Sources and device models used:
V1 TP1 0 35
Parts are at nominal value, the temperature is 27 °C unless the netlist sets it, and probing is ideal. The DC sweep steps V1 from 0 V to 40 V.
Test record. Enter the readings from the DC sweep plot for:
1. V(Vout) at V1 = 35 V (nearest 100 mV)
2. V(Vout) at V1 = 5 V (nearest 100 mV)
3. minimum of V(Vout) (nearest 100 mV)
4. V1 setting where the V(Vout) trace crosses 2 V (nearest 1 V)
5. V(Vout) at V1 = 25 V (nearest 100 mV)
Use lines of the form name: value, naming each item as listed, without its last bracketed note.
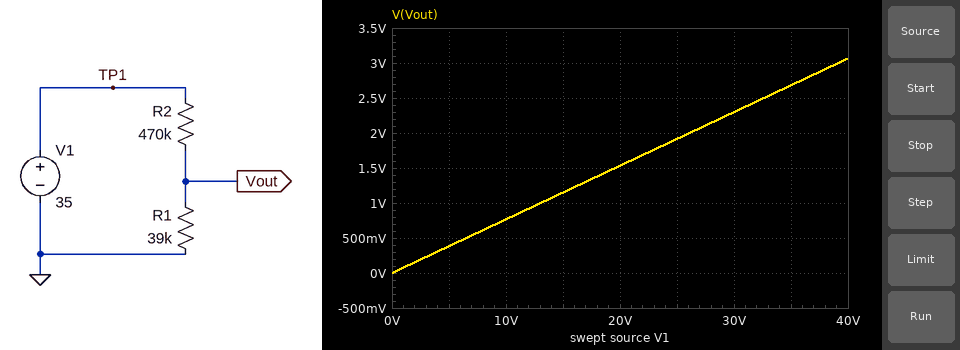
V(Vout) at V1 = 35 V: 2.7 V
V(Vout) at V1 = 5 V: 400 mV
minimum of V(Vout): 0 V
V1 setting where the V(Vout) trace crosses 2 V: 26 V
V(Vout) at V1 = 25 V: 1.9 V
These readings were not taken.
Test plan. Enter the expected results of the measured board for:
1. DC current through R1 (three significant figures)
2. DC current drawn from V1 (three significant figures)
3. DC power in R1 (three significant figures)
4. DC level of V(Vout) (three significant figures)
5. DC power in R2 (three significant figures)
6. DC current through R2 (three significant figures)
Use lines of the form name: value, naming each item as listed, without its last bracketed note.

DC current through R1: 68.8 µA
DC current drawn from V1: 68.8 µA
DC power in R1: 184 µW
DC level of V(Vout): 2.68 V
DC power in R2: 2.22 mW
DC current through R2: 68.8 µA
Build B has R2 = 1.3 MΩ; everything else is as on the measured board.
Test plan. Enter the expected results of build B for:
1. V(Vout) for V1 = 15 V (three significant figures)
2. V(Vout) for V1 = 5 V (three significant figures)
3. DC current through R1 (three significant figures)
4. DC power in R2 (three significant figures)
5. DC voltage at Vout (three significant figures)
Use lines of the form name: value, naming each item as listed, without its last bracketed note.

V(Vout) for V1 = 15 V: 437 mV
V(Vout) for V1 = 5 V: 146 mV
DC current through R1: 26.1 µA
DC power in R2: 888 µW
DC voltage at Vout: 1.02 V
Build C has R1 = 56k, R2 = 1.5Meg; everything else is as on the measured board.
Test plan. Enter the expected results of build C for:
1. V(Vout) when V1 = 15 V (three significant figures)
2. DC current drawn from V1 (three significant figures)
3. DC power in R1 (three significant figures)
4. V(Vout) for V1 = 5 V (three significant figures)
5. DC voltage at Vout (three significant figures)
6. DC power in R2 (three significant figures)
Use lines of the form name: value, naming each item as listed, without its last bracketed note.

V(Vout) when V1 = 15 V: 540 mV
DC current drawn from V1: 22.5 µA
DC power in R1: 28.3 µW
V(Vout) for V1 = 5 V: 180 mV
DC voltage at Vout: 1.26 V
DC power in R2: 759 µW
